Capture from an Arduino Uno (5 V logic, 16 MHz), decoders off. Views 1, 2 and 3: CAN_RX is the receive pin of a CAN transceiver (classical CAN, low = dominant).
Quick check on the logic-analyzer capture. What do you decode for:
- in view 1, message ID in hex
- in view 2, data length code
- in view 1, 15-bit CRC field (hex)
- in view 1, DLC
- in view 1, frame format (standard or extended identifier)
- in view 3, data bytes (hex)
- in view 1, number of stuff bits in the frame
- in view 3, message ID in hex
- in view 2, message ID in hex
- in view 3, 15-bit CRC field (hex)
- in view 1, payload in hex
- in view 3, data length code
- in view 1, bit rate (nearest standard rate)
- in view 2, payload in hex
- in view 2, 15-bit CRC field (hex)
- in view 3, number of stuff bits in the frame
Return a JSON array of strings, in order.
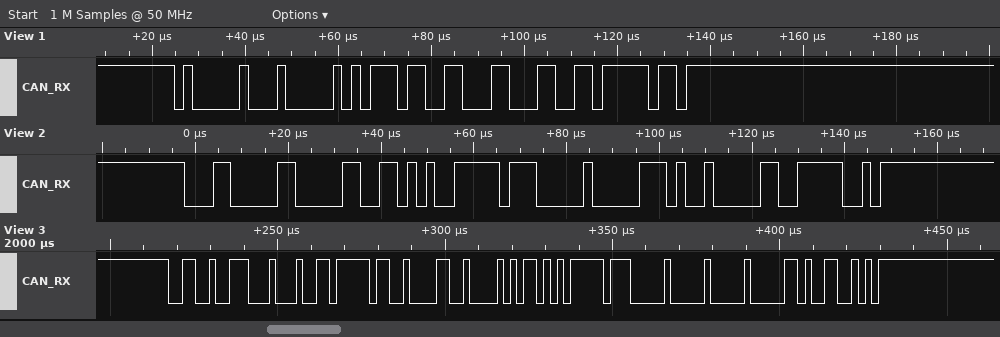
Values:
["0x402", "4", "0x19BF", "2", "standard", "9B F9 0C 85 6A FF 00 00", "3", "0x327", "0x182", "0x0532", "EC C6", "8", "500 kbit/s", "D4 FF 00 34", "0x413E", "6"]
